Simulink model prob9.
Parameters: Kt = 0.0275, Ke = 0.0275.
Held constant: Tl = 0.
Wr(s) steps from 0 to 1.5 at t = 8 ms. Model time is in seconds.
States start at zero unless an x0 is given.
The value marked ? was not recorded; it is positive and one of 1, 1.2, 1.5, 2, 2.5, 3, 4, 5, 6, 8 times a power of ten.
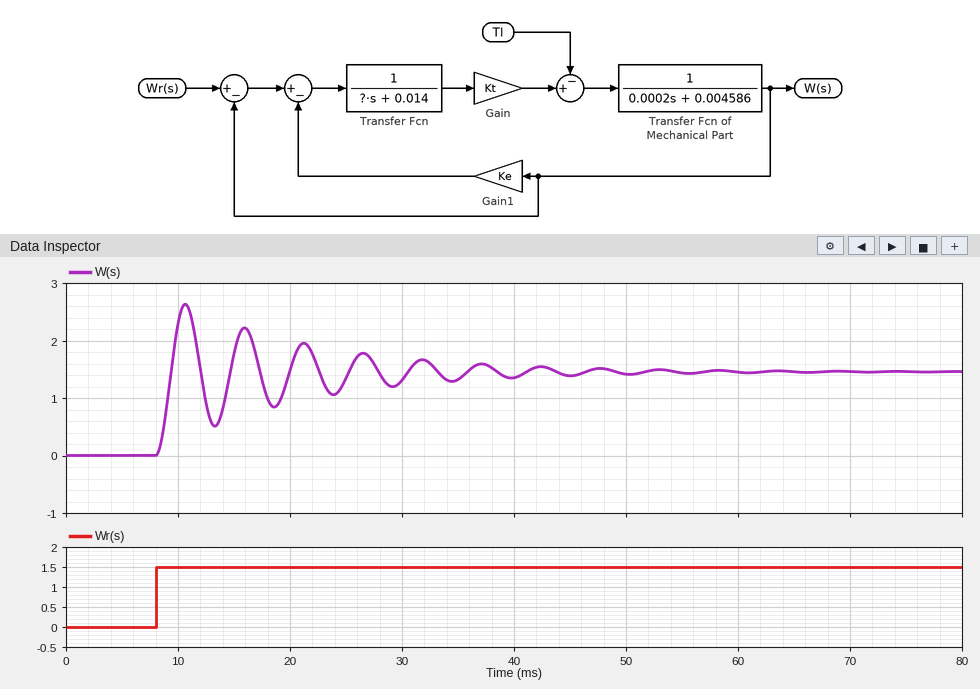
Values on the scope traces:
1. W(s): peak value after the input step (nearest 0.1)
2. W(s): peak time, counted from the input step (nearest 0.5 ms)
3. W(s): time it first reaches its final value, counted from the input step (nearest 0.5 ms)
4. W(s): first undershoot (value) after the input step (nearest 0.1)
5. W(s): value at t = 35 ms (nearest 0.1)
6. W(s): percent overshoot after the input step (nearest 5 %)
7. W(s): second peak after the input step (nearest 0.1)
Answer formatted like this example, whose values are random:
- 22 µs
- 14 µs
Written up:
- 2.6
- 2.5 ms
- 1.5 ms
- 0.5
- 1.3
- 80 %
- 2.2
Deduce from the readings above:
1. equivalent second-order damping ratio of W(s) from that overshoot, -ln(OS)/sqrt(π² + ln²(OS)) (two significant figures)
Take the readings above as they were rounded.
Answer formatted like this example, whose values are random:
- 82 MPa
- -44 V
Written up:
- 0.071
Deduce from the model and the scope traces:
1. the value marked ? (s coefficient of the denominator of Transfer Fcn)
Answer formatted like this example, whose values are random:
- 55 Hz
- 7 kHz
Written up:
- 0.0001
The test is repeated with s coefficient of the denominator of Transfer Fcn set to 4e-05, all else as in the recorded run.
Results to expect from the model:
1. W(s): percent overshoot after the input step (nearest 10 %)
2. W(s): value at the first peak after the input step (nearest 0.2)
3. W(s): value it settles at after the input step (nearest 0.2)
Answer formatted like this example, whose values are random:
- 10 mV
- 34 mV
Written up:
- 70 %
- 2.6
- 1.4
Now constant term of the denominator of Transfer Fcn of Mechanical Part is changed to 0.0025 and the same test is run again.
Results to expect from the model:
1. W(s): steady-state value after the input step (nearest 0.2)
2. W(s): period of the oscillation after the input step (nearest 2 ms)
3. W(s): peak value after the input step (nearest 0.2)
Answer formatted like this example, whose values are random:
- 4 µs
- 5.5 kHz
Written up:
- 1.4
- 6 ms
- 2.6
